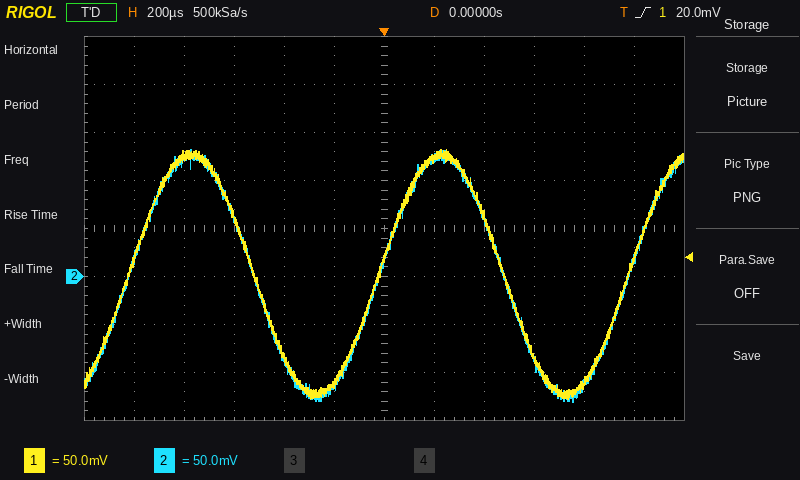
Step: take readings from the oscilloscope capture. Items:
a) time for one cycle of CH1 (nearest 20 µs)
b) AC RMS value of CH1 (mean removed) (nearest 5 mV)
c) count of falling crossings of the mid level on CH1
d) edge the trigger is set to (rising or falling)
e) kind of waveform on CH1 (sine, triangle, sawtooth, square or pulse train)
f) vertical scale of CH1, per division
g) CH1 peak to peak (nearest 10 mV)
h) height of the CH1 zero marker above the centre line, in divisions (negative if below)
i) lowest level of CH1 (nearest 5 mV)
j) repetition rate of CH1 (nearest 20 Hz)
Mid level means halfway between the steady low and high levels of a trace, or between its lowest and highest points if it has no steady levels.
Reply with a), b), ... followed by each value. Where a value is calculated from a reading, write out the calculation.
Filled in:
a) 1.00 ms
b) 260 mV / (2√2) ≈ 91.9 mV, so 90 mV to the nearest 5 mV
c) 2
d) rising
e) sine
f) 50 mV
g) 260 mV
h) -1.0 div
i) -130 mV
j) 1 / 1.00 ms ≈ 1.00 kHz
